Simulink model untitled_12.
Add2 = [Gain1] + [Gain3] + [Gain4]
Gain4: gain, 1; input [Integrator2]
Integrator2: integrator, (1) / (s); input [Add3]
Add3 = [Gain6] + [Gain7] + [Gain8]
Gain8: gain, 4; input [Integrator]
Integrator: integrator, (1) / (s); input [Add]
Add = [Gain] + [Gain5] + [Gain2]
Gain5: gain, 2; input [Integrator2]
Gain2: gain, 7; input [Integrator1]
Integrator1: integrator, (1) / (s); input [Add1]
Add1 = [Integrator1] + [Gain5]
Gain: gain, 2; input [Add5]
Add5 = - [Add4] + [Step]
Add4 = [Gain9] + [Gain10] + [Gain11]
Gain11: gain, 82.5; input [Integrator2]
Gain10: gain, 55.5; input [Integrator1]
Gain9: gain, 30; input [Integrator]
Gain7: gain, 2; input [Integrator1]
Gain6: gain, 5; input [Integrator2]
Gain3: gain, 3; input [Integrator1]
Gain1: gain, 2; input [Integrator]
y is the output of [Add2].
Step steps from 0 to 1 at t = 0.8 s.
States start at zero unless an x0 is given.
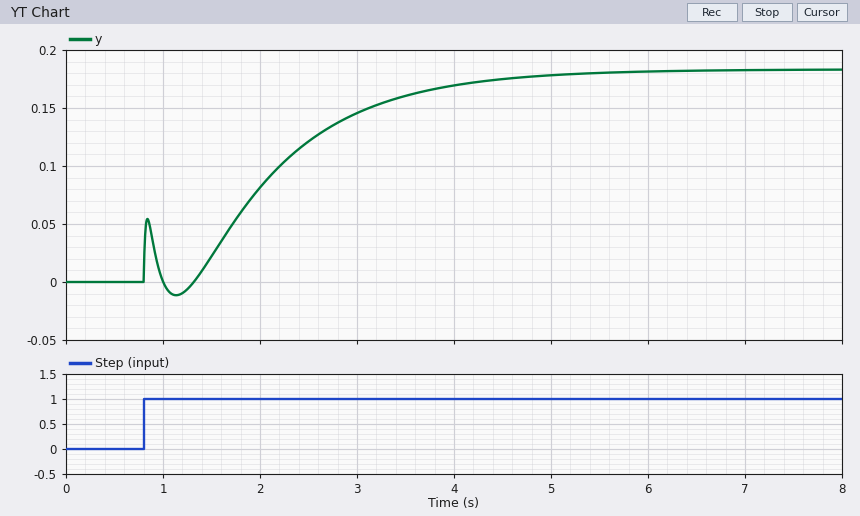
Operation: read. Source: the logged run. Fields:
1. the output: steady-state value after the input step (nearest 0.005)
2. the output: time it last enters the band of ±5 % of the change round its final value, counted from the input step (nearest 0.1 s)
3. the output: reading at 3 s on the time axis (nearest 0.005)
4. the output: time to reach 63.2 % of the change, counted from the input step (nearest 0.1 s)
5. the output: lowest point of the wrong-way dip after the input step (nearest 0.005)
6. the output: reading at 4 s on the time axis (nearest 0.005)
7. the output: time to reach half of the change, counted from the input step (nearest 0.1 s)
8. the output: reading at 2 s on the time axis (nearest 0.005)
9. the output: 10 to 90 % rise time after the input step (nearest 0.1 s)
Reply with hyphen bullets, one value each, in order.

- 0.185
- 3.6 s
- 0.145
- 1.6 s
- -0.010
- 0.170
- 1.3 s
- 0.080
- 2.9 s
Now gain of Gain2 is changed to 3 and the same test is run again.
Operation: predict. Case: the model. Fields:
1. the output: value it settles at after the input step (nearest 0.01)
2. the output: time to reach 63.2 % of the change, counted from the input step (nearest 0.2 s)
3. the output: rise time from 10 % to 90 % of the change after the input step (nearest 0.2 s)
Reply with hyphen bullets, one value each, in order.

- 0.16
- 1.4 s
- 2.6 s
